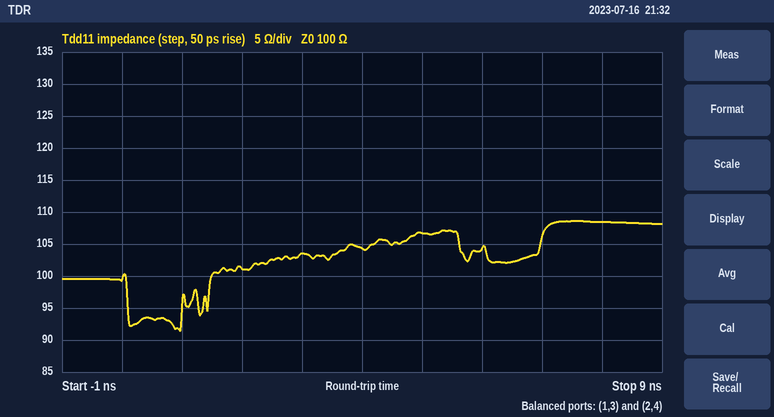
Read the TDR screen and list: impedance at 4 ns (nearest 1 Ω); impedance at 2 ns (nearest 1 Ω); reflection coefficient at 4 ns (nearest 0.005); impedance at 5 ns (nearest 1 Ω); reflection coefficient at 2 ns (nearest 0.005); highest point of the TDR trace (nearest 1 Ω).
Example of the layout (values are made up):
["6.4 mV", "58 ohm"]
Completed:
["104 Ω", "101 Ω", "+0.020", "107 Ω", "+0.005", "109 Ω"]
